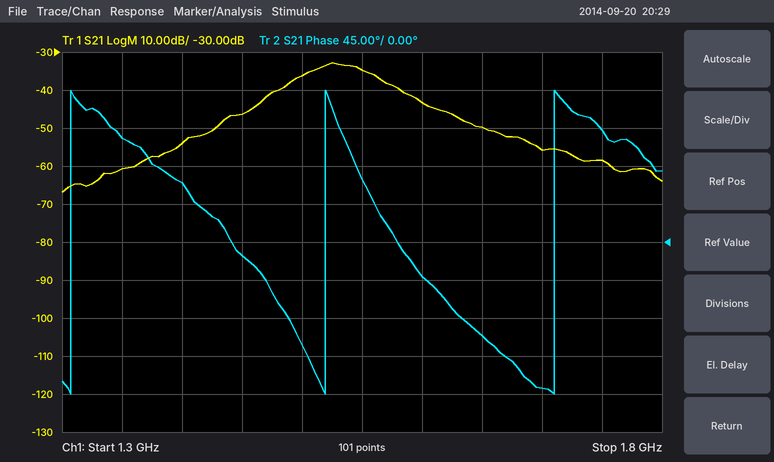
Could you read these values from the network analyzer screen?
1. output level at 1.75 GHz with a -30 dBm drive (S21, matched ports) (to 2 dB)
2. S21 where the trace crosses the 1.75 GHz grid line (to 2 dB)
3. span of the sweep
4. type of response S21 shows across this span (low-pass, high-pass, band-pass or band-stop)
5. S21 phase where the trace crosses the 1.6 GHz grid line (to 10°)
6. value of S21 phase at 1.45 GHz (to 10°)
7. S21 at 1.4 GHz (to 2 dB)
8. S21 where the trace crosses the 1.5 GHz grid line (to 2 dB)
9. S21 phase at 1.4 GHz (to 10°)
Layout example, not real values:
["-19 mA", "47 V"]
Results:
["-88 dBm", "-58 dB", "500 MHz", "band-pass", "-40°", "-20°", "-54 dB", "-36 dB", "70°"]
